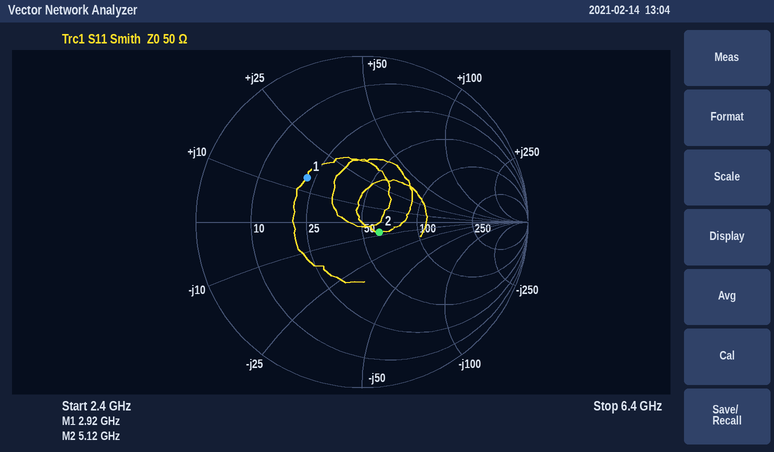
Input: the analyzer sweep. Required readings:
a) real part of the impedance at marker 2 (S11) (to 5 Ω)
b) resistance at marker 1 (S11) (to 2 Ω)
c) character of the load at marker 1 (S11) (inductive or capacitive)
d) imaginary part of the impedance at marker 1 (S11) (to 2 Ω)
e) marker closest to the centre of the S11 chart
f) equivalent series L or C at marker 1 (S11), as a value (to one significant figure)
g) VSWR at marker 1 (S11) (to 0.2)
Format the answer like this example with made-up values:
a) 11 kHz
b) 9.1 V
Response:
a) 60 Ω
b) 22 Ω
c) inductive
d) +14 Ω
e) marker 2
f) 800 pH
g) 2.4
